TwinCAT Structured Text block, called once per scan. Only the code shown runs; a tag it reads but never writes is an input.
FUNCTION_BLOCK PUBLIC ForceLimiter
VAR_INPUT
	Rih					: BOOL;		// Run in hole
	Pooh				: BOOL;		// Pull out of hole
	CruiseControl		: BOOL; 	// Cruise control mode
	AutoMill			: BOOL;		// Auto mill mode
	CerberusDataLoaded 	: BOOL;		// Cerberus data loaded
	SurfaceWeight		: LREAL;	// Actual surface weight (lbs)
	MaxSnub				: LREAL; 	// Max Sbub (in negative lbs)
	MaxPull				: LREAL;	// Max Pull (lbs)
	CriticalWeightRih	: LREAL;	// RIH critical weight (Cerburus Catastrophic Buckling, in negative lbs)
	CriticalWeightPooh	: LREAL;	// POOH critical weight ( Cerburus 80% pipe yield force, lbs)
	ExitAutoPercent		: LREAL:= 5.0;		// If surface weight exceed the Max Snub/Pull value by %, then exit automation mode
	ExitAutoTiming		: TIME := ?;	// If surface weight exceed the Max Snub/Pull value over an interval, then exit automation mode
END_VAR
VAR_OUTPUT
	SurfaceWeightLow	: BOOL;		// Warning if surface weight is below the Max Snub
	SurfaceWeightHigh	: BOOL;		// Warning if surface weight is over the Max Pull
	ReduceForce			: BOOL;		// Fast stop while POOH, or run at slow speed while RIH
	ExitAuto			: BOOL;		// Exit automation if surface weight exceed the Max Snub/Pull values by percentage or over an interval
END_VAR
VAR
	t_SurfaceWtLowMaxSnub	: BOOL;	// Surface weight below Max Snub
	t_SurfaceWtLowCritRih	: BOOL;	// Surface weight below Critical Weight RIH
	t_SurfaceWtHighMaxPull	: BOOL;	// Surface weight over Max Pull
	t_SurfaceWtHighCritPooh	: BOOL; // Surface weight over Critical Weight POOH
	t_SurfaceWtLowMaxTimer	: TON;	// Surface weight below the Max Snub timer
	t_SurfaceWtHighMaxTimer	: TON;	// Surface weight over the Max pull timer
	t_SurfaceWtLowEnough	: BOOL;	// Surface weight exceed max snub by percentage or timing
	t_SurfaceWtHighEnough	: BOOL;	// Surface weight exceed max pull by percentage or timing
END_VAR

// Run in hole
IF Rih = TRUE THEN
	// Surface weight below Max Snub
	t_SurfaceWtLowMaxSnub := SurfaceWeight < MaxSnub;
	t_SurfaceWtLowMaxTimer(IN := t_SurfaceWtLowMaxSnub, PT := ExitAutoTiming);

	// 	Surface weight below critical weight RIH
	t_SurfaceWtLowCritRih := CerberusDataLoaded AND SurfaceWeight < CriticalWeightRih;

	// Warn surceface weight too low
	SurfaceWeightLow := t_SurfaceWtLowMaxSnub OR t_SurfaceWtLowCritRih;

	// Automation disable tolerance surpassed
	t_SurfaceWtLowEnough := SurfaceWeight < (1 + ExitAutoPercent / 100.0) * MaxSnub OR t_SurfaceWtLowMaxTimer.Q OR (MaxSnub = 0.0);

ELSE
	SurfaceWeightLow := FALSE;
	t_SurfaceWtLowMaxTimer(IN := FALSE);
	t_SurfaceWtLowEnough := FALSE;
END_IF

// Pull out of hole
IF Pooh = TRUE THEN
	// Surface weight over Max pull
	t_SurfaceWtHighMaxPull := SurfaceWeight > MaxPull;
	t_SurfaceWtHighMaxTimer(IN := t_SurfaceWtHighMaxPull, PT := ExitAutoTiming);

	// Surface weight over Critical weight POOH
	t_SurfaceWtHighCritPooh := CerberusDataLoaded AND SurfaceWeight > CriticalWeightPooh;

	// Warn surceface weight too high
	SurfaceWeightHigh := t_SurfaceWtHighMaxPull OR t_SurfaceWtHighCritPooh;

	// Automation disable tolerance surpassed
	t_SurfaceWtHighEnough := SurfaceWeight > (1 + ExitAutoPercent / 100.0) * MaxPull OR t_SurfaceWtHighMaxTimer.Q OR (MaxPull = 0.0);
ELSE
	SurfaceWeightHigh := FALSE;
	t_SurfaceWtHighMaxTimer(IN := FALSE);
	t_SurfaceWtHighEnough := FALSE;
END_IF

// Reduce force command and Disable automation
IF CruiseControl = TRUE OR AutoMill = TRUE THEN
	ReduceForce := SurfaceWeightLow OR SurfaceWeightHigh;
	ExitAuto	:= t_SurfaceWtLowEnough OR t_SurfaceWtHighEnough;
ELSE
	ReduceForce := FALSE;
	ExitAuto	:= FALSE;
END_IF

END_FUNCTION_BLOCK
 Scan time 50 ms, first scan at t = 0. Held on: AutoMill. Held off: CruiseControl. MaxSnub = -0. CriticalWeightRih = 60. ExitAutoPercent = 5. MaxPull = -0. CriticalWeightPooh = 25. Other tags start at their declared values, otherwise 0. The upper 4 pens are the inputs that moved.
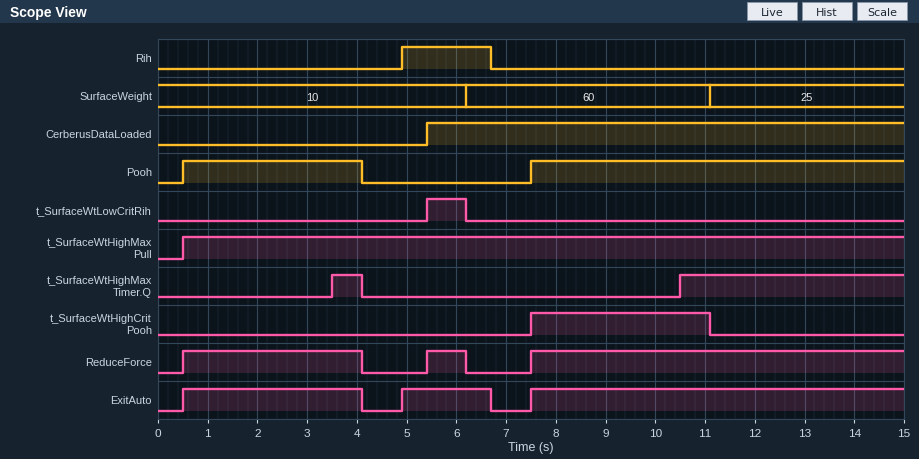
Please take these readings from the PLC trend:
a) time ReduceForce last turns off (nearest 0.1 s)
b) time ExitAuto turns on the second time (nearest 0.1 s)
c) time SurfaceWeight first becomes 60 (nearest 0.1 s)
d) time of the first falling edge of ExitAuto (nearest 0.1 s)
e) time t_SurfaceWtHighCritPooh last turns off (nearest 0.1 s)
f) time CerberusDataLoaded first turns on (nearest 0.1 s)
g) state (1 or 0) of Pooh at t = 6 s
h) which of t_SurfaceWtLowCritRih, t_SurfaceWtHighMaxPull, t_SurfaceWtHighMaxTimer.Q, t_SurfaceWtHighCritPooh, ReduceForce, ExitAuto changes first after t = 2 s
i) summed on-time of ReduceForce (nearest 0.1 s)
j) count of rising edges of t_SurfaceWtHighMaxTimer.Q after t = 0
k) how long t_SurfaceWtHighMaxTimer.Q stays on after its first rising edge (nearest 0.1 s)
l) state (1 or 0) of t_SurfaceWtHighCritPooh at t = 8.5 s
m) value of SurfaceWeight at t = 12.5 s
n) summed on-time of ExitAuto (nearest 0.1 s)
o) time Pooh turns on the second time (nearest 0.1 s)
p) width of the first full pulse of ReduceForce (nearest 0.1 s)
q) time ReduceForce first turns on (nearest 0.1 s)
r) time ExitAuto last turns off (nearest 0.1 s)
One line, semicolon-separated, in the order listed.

6.2 s; 4.9 s; 6.2 s; 4.1 s; 11.1 s; 5.4 s; 0; t_SurfaceWtHighMaxTimer.Q; 11.9 s; 2; 0.6 s; 1; 25; 12.9 s; 7.5 s; 3.6 s; 0.5 s; 6.7 s
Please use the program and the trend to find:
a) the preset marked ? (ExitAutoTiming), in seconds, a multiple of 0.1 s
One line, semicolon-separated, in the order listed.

3.0 s
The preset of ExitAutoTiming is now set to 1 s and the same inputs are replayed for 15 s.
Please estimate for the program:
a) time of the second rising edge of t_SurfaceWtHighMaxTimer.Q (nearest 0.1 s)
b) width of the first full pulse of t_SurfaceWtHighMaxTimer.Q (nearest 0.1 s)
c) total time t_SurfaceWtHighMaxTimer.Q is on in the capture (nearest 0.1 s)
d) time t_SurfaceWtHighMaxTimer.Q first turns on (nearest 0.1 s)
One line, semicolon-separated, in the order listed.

8.5 s; 2.6 s; 9.1 s; 1.5 s
